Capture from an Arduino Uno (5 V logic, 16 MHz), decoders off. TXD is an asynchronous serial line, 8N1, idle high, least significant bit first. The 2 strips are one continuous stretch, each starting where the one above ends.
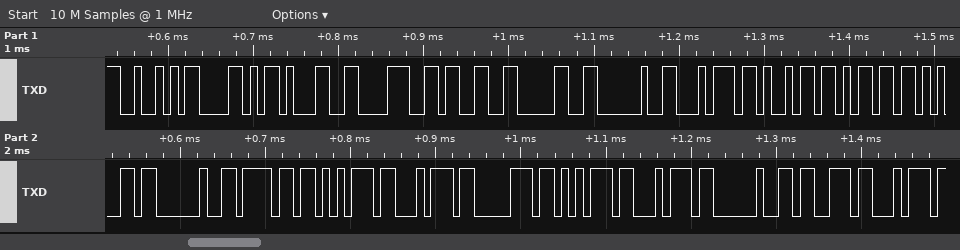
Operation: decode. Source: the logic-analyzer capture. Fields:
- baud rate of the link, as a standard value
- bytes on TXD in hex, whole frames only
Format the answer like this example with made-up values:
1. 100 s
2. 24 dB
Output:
1. 115200 baud
2. 0x52 0x58 0x31 0x38 0x33 0x30 0x20 0x74 0x69 0x6D 0x65 0x20 0x6F 0x75 0x74 0x70 0x75 0x74 0x20 0x73 0x74
